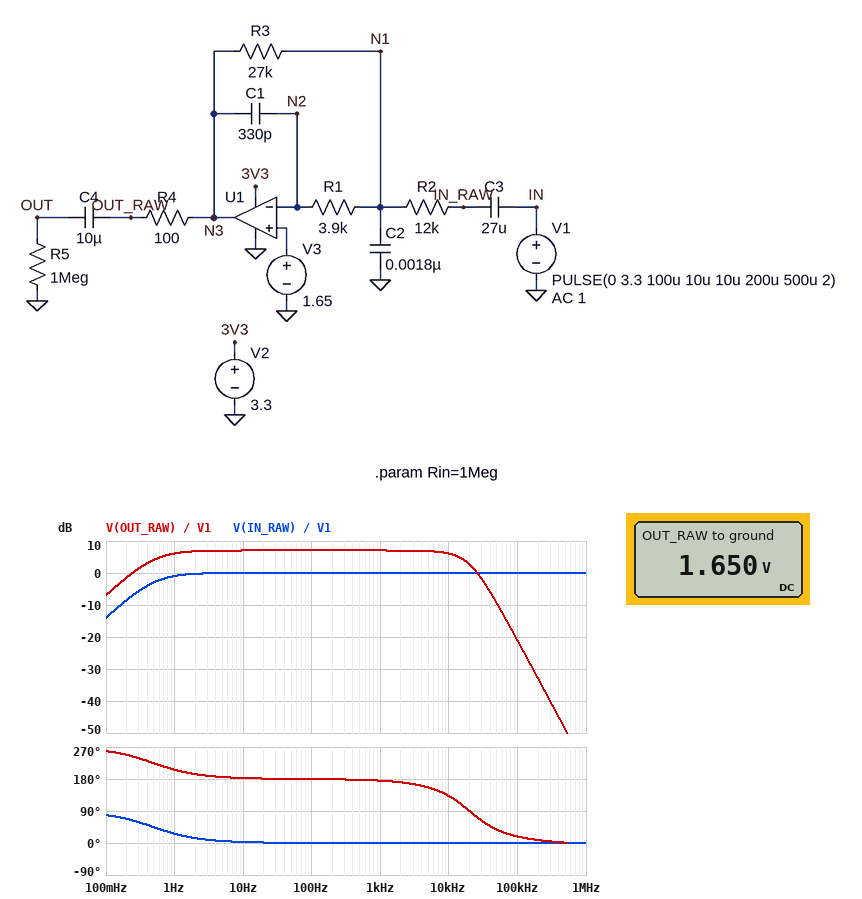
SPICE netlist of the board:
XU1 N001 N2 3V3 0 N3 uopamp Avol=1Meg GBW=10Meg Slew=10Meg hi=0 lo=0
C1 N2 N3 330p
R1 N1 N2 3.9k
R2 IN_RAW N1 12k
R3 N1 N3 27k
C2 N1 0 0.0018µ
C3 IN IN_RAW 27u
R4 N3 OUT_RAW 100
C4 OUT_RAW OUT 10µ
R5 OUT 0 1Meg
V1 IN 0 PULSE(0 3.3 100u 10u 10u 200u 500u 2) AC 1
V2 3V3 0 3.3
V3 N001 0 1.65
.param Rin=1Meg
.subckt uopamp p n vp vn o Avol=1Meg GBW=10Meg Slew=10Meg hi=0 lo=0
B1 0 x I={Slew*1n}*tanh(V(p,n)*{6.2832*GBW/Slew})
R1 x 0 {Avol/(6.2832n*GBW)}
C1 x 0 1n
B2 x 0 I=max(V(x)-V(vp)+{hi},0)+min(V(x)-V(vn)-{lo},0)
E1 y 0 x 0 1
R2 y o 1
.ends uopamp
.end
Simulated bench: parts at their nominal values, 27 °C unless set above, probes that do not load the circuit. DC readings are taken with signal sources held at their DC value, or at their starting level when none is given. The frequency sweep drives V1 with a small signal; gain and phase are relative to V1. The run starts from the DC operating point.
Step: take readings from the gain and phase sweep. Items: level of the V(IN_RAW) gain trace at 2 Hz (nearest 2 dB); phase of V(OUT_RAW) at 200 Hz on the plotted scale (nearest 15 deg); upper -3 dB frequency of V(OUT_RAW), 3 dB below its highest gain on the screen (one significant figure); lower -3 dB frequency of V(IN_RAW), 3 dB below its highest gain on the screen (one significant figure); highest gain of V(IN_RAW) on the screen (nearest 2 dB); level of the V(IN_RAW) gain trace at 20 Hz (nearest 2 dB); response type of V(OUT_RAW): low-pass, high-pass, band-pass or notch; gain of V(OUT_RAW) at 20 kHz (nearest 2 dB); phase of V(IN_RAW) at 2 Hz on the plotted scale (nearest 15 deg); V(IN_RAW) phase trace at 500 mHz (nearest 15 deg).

0 dB
180 deg
20 kHz
500 mHz
0 dB
0 dB
band-pass
2 dB
15 deg
45 deg
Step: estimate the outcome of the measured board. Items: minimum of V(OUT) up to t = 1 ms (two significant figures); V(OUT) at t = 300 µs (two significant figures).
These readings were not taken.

-1.7 V
-1.7 V
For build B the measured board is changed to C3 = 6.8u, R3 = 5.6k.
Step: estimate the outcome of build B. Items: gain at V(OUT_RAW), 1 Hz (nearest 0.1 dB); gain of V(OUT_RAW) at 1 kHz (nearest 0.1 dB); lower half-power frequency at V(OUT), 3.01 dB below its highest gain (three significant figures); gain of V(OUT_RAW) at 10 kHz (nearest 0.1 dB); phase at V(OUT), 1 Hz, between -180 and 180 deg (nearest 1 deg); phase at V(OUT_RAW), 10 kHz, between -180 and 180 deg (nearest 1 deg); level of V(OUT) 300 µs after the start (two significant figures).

-13.4 dB
-6.6 dB
2.60 Hz
-6.4 dB
-116 deg
166 deg
-1.5 V
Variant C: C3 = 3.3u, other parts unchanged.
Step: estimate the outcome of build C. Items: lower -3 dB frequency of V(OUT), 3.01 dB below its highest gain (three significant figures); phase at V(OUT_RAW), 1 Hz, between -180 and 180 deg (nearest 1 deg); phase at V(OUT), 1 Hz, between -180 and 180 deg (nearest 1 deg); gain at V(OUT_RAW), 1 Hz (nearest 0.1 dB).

4.02 Hz
-104 deg
-103 deg
-5.3 dB
